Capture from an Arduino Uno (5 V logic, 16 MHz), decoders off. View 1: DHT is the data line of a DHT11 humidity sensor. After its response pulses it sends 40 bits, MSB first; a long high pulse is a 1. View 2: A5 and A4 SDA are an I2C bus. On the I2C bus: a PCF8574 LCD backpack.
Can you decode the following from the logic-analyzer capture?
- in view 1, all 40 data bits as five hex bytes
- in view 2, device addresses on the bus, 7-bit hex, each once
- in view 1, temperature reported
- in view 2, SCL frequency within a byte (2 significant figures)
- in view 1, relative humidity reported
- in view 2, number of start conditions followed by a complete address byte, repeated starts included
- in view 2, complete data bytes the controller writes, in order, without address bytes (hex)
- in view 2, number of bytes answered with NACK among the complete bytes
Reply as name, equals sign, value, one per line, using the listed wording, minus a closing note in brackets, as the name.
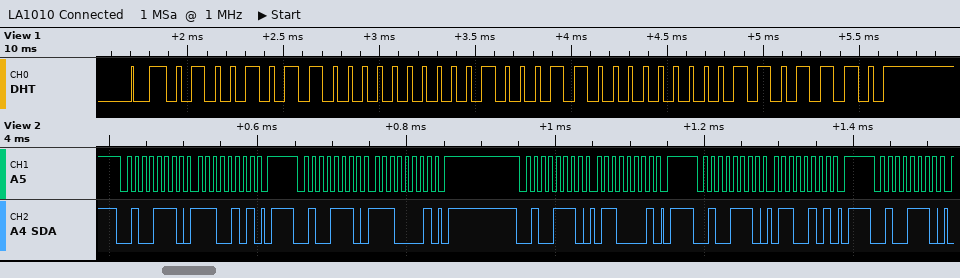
in view 1, all 40 data bits as five hex bytes = 4B 00 23 00 6E
in view 2, device addresses on the bus, 7-bit hex, each once = 0x27
in view 1, temperature reported = 35.0 °C
in view 2, SCL frequency within a byte = 100 kHz
in view 1, relative humidity reported = 75 %
in view 2, number of start conditions followed by a complete address byte, repeated starts included = 5
in view 2, complete data bytes the controller writes, in order, without address bytes = E5 E1 61 65
in view 2, number of bytes answered with NACK among the complete bytes = 0
